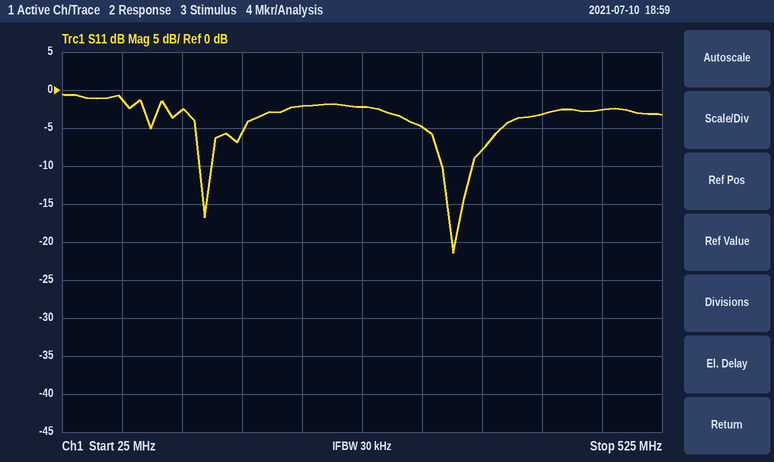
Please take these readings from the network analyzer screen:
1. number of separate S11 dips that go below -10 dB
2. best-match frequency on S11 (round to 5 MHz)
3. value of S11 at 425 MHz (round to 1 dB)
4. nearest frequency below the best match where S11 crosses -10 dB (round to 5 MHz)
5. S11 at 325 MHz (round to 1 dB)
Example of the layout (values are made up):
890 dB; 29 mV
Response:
2; 350 MHz; -3 dB; 340 MHz; -5 dB
